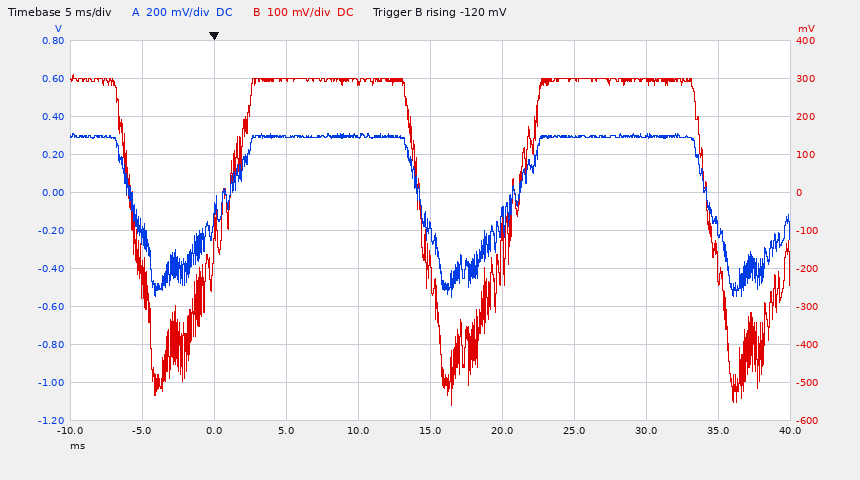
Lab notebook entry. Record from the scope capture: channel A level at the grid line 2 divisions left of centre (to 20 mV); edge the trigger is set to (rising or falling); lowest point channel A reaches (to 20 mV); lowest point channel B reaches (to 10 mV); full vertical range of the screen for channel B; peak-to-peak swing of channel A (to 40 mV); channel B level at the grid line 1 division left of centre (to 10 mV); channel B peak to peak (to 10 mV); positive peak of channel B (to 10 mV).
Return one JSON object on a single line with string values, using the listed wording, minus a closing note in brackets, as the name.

{"channel A level at the grid line 2 divisions left of centre": "300 mV", "edge the trigger is set to": "rising", "lowest point channel A reaches": "-560 mV", "lowest point channel B reaches": "-560 mV", "full vertical range of the screen for channel B": "1 V", "peak-to-peak swing of channel A": "880 mV", "channel B level at the grid line 1 division left of centre": "290 mV", "channel B peak to peak": "870 mV", "positive peak of channel B": "310 mV"}
